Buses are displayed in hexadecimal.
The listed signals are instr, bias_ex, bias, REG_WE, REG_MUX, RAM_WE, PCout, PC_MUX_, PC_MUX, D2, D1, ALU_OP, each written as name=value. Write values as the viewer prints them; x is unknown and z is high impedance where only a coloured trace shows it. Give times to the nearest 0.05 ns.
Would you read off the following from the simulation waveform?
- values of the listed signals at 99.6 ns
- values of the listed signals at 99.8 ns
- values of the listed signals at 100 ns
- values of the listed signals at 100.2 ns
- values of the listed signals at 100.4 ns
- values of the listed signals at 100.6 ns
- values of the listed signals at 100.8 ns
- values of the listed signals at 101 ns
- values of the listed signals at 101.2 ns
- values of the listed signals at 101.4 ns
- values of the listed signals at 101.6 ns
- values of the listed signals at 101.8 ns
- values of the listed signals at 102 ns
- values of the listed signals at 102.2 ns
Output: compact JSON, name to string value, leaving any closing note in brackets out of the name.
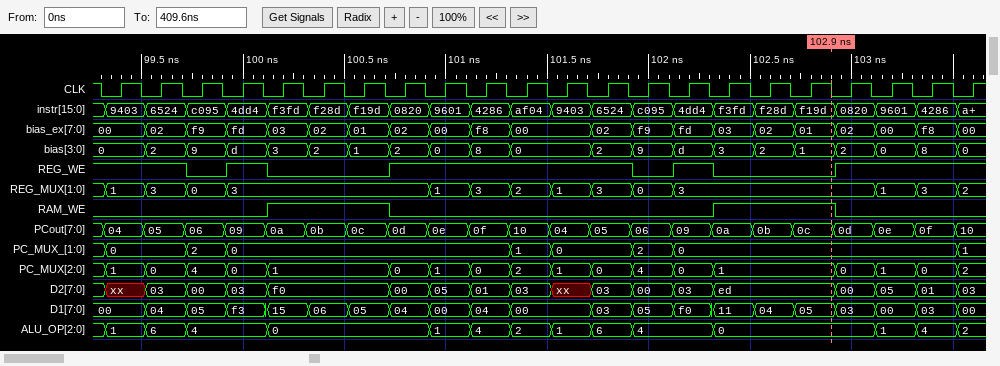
{"values of the listed signals at 99.6 ns": "instr=6524, bias_ex=02, bias=2, REG_WE=1, REG_MUX=3, RAM_WE=0, PCout=05, PC_MUX_=0, PC_MUX=0, D2=03, D1=04, ALU_OP=6", "values of the listed signals at 99.8 ns": "instr=c095, bias_ex=f9, bias=9, REG_WE=0, REG_MUX=0, RAM_WE=0, PCout=06, PC_MUX_=2, PC_MUX=4, D2=00, D1=05, ALU_OP=4", "values of the listed signals at 100 ns": "instr=4dd4, bias_ex=fd, bias=d, REG_WE=1, REG_MUX=3, RAM_WE=0, PCout=09, PC_MUX_=0, PC_MUX=0, D2=03, D1=f3, ALU_OP=4", "values of the listed signals at 100.2 ns": "instr=f3fd, bias_ex=03, bias=3, REG_WE=0, REG_MUX=3, RAM_WE=1, PCout=0a, PC_MUX_=0, PC_MUX=1, D2=f0, D1=15, ALU_OP=0", "values of the listed signals at 100.4 ns": "instr=f28d, bias_ex=02, bias=2, REG_WE=0, REG_MUX=3, RAM_WE=1, PCout=0b, PC_MUX_=0, PC_MUX=1, D2=f0, D1=06, ALU_OP=0", "values of the listed signals at 100.6 ns": "instr=f19d, bias_ex=01, bias=1, REG_WE=0, REG_MUX=3, RAM_WE=1, PCout=0c, PC_MUX_=0, PC_MUX=1, D2=f0, D1=05, ALU_OP=0", "values of the listed signals at 100.8 ns": "instr=0820, bias_ex=02, bias=2, REG_WE=1, REG_MUX=3, RAM_WE=0, PCout=0d, PC_MUX_=0, PC_MUX=0, D2=00, D1=04, ALU_OP=0", "values of the listed signals at 101 ns": "instr=9601, bias_ex=00, bias=0, REG_WE=1, REG_MUX=1, RAM_WE=0, PCout=0e, PC_MUX_=0, PC_MUX=1, D2=05, D1=00, ALU_OP=1", "values of the listed signals at 101.2 ns": "instr=4286, bias_ex=f8, bias=8, REG_WE=1, REG_MUX=3, RAM_WE=0, PCout=0f, PC_MUX_=0, PC_MUX=0, D2=01, D1=04, ALU_OP=4", "values of the listed signals at 101.4 ns": "instr=af04, bias_ex=00, bias=0, REG_WE=1, REG_MUX=2, RAM_WE=0, PCout=10, PC_MUX_=1, PC_MUX=2, D2=03, D1=00, ALU_OP=2", "values of the listed signals at 101.6 ns": "instr=9403, bias_ex=00, bias=0, REG_WE=1, REG_MUX=1, RAM_WE=0, PCout=04, PC_MUX_=0, PC_MUX=1, D2=xx, D1=00, ALU_OP=1", "values of the listed signals at 101.8 ns": "instr=6524, bias_ex=02, bias=2, REG_WE=1, REG_MUX=3, RAM_WE=0, PCout=05, PC_MUX_=0, PC_MUX=0, D2=03, D1=03, ALU_OP=6", "values of the listed signals at 102 ns": "instr=c095, bias_ex=f9, bias=9, REG_WE=0, REG_MUX=0, RAM_WE=0, PCout=06, PC_MUX_=2, PC_MUX=4, D2=00, D1=05, ALU_OP=4", "values of the listed signals at 102.2 ns": "instr=4dd4, bias_ex=fd, bias=d, REG_WE=1, REG_MUX=3, RAM_WE=0, PCout=09, PC_MUX_=0, PC_MUX=0, D2=03, D1=f0, ALU_OP=4"}
